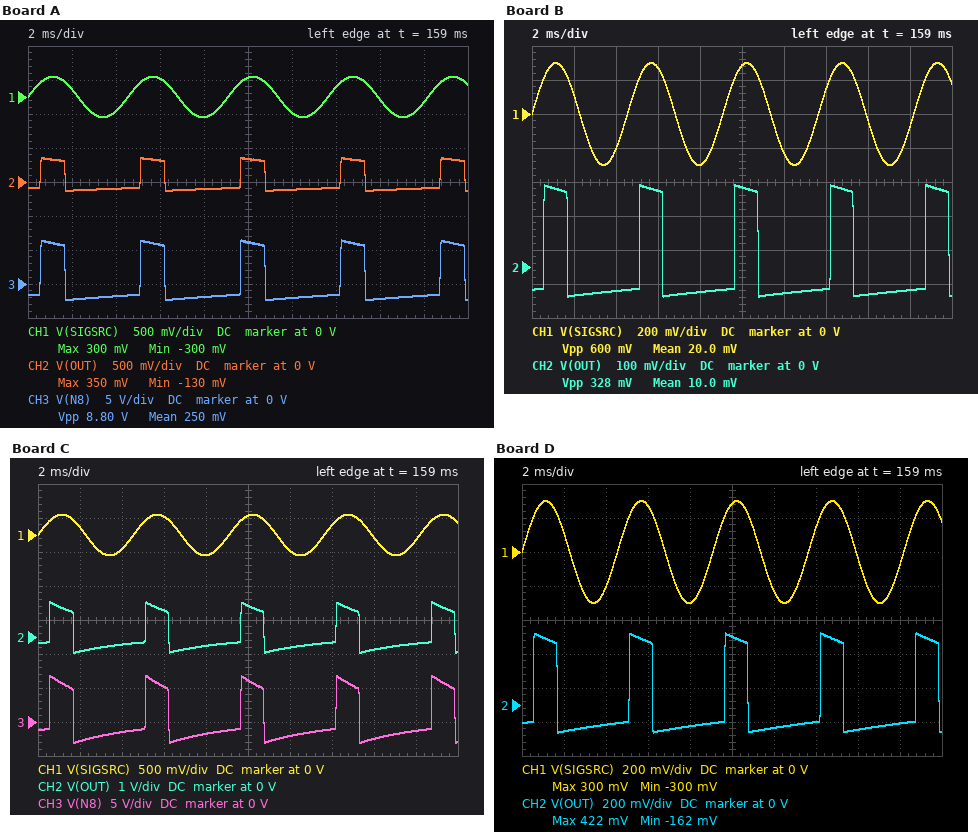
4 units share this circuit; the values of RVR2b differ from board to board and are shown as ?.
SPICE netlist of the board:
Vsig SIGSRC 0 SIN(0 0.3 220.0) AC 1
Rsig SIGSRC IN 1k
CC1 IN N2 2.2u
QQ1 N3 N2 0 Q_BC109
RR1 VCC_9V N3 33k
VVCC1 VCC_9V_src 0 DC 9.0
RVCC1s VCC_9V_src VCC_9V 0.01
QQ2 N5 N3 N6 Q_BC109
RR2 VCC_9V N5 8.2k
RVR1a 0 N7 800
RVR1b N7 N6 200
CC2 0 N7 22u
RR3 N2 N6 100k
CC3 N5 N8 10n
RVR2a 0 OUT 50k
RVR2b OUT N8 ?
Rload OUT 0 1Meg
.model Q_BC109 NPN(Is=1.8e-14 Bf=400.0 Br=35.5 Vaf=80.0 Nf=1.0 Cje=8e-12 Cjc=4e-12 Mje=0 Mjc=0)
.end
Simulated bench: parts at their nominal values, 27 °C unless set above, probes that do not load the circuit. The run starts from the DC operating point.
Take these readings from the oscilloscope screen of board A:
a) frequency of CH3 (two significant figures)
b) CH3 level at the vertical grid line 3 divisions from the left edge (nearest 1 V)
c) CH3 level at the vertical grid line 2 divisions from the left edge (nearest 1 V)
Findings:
220 Hz
6 V
-2 V
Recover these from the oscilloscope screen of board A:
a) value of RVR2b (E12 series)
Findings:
820 kΩ
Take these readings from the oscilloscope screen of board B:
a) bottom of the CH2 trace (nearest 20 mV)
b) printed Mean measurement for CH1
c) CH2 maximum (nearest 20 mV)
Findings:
-80 mV
20.0 mV
240 mV
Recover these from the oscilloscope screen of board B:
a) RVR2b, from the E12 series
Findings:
1.2 MΩ
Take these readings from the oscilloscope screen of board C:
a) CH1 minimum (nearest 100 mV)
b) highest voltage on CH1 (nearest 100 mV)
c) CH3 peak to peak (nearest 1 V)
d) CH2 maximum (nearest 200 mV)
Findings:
-300 mV
300 mV
10 V
1.0 V
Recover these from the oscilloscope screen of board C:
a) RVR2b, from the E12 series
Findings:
270 kΩ
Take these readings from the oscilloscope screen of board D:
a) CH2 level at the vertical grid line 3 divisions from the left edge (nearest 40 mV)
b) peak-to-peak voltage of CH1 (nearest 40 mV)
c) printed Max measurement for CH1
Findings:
360 mV
600 mV
300 mV
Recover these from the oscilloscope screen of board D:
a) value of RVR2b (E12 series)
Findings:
680 kΩ
